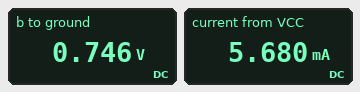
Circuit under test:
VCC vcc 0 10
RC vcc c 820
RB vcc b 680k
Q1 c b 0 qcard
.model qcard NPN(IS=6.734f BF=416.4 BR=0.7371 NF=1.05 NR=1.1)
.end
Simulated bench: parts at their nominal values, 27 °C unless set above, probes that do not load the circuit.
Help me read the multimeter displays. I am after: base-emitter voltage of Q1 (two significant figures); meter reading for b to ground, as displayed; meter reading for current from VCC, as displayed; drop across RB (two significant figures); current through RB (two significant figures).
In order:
750 mV
0.746 V
5.680 mA
9.3 V
14 µA
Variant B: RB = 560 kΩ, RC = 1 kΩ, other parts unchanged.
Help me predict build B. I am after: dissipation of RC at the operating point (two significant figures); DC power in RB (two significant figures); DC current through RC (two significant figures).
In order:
47 mW
150 µW
6.9 mA
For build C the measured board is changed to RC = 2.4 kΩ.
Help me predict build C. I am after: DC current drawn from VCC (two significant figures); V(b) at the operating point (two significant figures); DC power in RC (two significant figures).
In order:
4.1 mA
740 mV
40 mW
